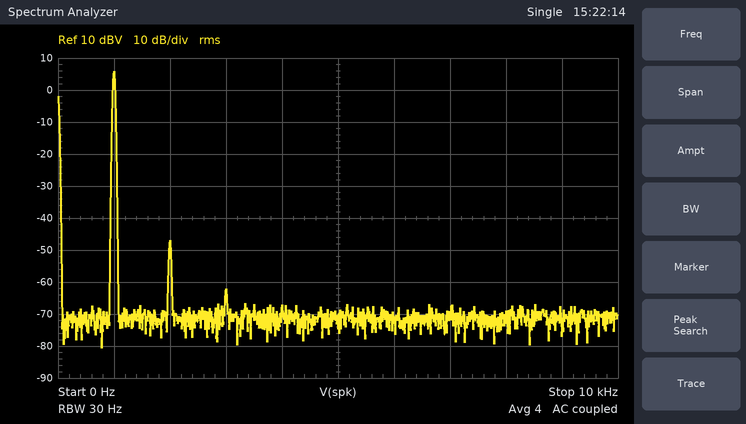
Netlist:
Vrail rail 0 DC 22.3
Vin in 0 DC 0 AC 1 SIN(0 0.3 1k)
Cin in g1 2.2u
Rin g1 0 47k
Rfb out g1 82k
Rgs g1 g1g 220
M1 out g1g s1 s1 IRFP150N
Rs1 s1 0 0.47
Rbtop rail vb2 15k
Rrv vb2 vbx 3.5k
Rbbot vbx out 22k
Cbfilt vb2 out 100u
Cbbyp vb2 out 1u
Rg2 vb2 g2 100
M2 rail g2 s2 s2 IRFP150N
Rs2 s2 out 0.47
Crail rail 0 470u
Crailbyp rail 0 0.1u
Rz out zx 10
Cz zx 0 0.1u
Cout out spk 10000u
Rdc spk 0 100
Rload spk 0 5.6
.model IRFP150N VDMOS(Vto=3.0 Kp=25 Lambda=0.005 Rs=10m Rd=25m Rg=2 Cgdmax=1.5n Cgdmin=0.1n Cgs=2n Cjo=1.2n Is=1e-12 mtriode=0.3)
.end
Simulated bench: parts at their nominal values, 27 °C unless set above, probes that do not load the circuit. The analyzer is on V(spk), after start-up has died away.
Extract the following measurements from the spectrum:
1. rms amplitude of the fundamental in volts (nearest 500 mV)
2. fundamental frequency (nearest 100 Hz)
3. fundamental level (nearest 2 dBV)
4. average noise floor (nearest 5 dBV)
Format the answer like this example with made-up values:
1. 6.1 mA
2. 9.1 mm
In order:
1. 2.0 V
2. 1.0 kHz
3. 6 dBV
4. -70 dBV
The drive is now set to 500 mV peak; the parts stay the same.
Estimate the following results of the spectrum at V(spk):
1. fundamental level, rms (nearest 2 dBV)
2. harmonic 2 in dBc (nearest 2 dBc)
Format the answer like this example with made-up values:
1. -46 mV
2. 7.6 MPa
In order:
1. 10 dBV
2. -48 dBc
